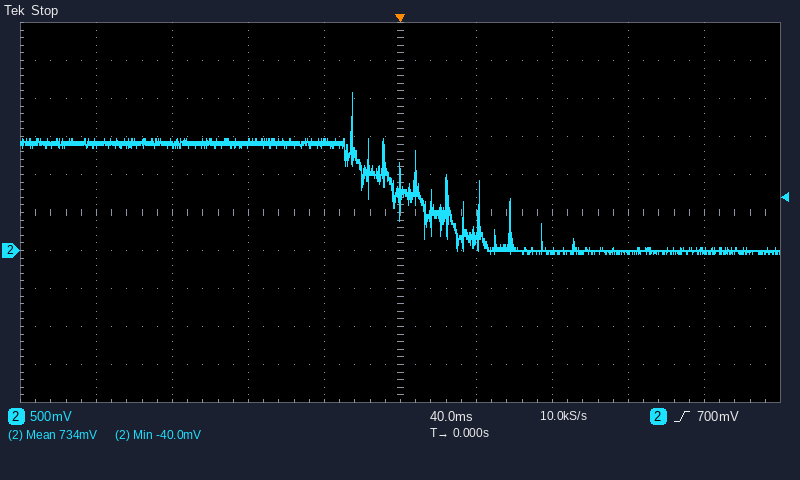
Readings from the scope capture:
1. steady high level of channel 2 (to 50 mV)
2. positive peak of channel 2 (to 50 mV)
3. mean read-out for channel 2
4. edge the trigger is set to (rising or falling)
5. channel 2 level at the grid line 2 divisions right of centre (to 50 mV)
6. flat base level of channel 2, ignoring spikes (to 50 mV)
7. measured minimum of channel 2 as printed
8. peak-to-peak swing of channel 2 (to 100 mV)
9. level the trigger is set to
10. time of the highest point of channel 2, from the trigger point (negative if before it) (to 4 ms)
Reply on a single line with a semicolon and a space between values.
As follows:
1.40 V; 2.10 V; 734 mV; rising; 0 mV; 0 mV; -40.0 mV; 2.10 V; 700 mV; -24 ms
